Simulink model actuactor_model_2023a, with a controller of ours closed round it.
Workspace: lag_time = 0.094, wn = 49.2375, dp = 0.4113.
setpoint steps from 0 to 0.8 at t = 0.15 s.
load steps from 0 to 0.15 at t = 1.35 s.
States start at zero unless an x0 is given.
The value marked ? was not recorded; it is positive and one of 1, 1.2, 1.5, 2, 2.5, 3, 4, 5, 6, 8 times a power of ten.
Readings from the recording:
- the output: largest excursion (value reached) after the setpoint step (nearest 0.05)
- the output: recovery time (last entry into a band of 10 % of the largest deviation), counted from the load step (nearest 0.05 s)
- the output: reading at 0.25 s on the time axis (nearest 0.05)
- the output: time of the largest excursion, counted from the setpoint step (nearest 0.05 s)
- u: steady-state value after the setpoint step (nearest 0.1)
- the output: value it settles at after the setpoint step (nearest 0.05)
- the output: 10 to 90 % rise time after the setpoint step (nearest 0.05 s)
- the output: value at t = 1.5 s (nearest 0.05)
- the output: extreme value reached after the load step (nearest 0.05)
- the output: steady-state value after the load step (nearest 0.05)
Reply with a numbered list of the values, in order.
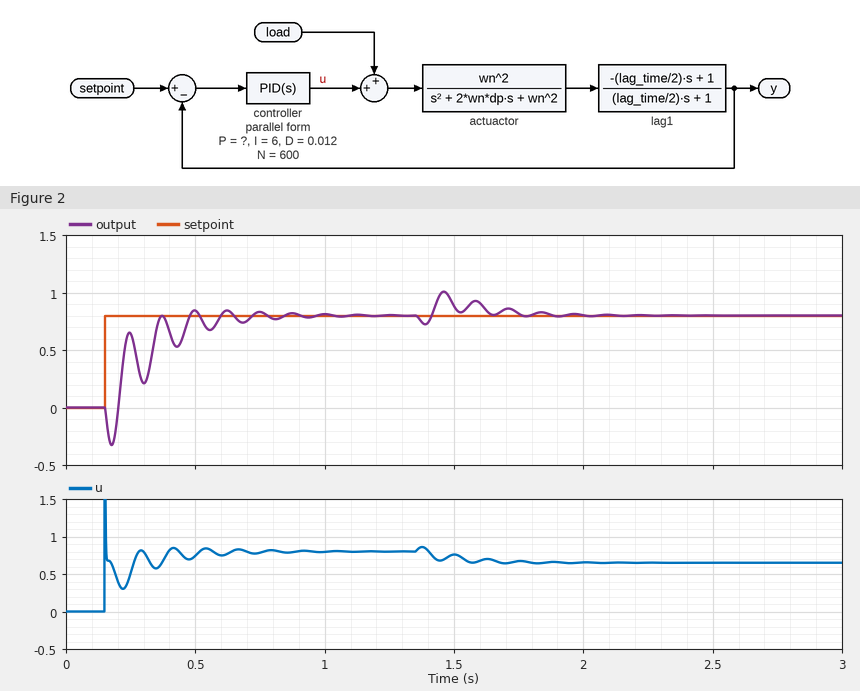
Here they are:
1. 0.85
2. 0.50 s
3. 0.65
4. 0.35 s
5. 0.8
6. 0.80
7. 0.15 s
8. 0.90
9. 1.00
10. 0.80
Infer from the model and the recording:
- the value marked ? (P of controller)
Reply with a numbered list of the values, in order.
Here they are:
1. 0.4
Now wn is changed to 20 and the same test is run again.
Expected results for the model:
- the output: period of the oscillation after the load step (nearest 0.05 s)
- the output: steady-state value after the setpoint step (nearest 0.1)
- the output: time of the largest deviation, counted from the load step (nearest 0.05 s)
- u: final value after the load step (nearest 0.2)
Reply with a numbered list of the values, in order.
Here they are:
1. 0.35 s
2. 0.8
3. 0.20 s
4. 0.6
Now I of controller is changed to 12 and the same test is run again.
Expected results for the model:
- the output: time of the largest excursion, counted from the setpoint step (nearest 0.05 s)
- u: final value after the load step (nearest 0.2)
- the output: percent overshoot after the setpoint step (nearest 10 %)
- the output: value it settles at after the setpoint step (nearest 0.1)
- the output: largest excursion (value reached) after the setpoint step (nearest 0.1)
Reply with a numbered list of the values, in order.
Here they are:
1. 0.25 s
2. 0.6
3. 30 %
4. 0.8
5. 1.0
